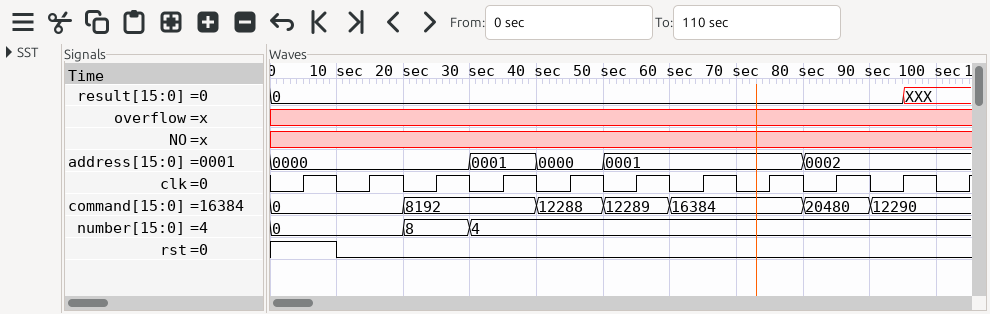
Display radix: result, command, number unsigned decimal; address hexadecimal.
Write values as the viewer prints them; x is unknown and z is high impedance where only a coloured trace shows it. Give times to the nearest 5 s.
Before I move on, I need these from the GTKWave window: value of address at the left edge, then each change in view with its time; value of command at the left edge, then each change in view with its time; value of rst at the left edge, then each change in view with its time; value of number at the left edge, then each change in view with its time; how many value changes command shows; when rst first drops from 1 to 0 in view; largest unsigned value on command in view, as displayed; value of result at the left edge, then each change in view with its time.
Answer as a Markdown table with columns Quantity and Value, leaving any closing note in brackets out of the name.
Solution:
| Quantity | Value |
|---|---|
| value of address at the left edge, then each change in view with its time | 0000, 0001 at 30 s, 0000 at 40 s, 0001 at 50 s, 0002 at 80 s |
| value of command at the left edge, then each change in view with its time | 0, 8192 at 20 s, 12288 at 40 s, 12289 at 50 s, 16384 at 60 s, 20480 at 80 s, 12290 at 90 s |
| value of rst at the left edge, then each change in view with its time | 1, 0 at 10 s |
| value of number at the left edge, then each change in view with its time | 0, 8 at 20 s, 4 at 30 s |
| how many value changes command shows | 6 |
| when rst first drops from 1 to 0 in view | 10 s |
| largest unsigned value on command in view, as displayed | 20480 |
| value of result at the left edge, then each change in view with its time | 0, XXX at 95 s |
